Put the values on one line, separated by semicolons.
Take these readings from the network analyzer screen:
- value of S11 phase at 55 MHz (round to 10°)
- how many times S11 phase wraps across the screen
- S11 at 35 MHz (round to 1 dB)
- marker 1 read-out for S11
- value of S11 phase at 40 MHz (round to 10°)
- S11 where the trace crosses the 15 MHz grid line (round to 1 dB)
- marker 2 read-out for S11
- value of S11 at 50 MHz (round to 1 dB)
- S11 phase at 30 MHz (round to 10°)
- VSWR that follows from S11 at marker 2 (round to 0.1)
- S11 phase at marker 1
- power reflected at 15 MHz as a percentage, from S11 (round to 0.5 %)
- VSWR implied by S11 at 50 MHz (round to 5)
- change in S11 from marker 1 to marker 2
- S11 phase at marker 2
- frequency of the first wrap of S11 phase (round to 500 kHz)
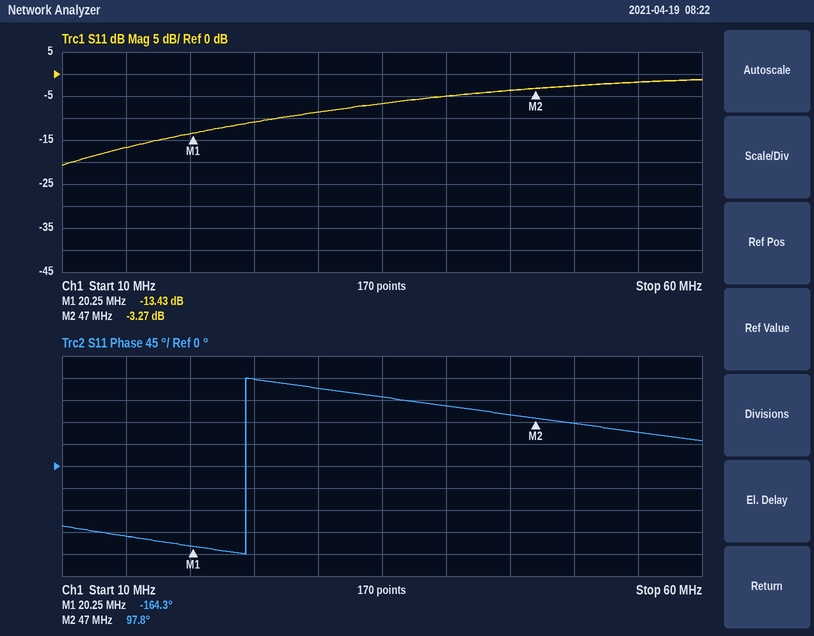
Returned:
70°; 1; -7 dB; -13.43 dB; 120°; -17 dB; -3.27 dB; -3 dB; 160°; 5.4; -164.3°; 2.0 %; 5; 10.16 dB; 97.8°; 24.5 MHz
